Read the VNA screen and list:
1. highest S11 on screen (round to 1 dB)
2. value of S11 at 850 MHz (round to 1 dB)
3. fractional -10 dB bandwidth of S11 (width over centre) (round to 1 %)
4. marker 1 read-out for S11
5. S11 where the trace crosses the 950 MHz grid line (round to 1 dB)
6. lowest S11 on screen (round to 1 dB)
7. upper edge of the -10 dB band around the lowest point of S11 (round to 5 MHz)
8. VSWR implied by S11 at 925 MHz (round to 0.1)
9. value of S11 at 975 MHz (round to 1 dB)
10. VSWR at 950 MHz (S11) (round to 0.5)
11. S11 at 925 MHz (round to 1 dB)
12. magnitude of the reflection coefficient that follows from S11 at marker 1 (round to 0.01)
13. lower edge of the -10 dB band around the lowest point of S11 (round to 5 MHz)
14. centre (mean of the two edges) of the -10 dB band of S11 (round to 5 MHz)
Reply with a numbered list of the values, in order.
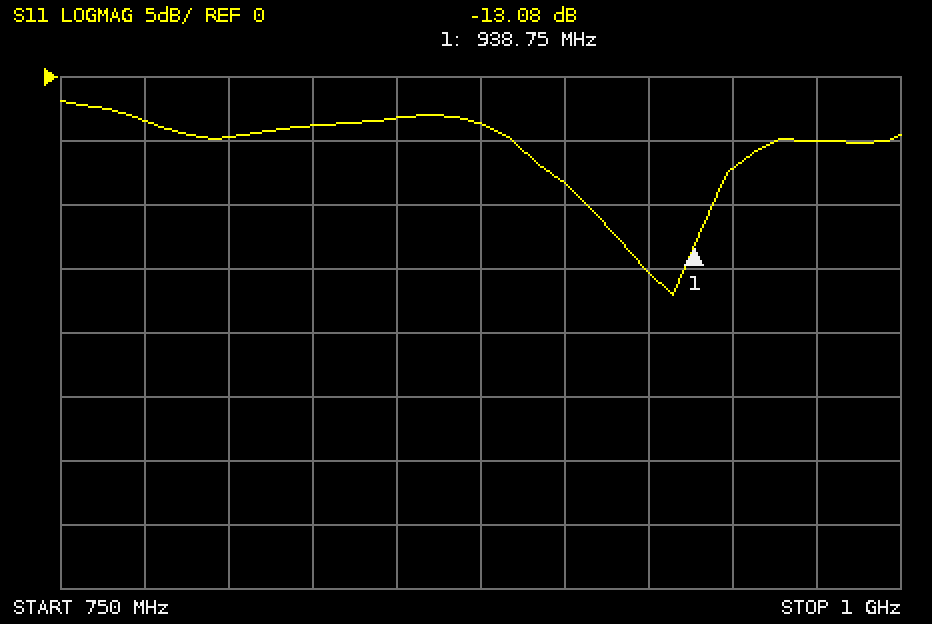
1. -2 dB
2. -3 dB
3. 4 %
4. -13.08 dB
5. -7 dB
6. -17 dB
7. 945 MHz
8. 1.4
9. -5 dB
10. 2.5
11. -15 dB
12. 0.22
13. 905 MHz
14. 925 MHz
